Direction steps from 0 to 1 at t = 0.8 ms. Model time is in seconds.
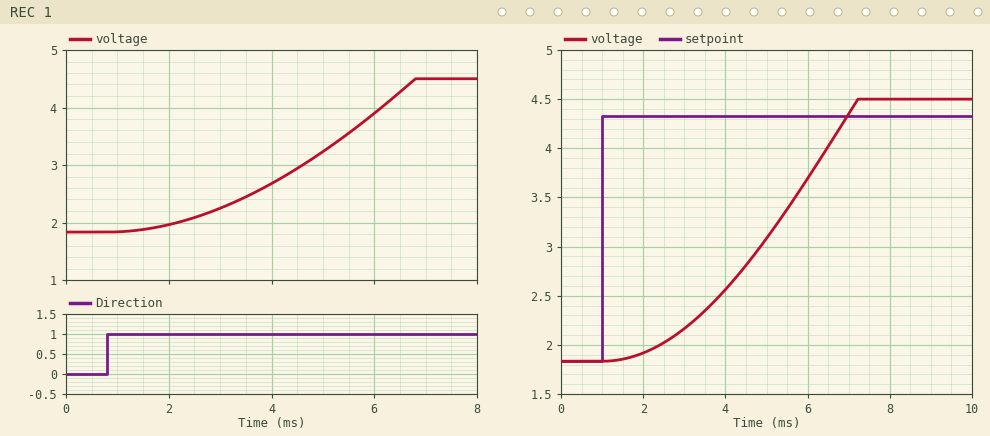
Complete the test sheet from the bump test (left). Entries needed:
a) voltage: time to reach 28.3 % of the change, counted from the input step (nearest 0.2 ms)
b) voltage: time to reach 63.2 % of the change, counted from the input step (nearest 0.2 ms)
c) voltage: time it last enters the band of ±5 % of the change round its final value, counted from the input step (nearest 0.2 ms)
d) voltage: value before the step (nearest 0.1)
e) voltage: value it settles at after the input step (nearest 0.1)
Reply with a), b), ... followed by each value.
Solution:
a) 3.0 ms
b) 4.6 ms
c) 5.8 ms
d) 1.8
e) 4.5
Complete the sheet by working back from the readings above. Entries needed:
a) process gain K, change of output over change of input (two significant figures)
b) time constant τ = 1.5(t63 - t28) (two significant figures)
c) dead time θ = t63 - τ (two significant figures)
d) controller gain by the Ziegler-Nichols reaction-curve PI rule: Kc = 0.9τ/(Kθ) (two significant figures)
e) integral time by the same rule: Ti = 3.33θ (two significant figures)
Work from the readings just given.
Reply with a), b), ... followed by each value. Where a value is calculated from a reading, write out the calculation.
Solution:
a) (4.5 - 1.8) / 1 = 2.7
b) 1.5 × (4.6 - 3) = 2.4 ms
c) 4.6 - 2.4 = 2.2 ms
d) 0.9 × 2.4 / (2.7 × 2.2) = 0.36
e) 3.33 × 2.2 = 7.3 ms
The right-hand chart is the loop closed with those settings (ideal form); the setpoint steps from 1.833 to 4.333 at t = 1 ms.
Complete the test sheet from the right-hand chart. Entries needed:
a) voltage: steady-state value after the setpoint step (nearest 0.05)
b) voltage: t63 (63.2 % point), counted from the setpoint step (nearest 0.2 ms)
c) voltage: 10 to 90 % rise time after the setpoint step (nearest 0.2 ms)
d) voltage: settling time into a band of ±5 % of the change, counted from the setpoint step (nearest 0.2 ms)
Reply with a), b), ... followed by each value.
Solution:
a) 4.50
b) 4.8 ms
c) 4.0 ms
d) 6.0 ms
